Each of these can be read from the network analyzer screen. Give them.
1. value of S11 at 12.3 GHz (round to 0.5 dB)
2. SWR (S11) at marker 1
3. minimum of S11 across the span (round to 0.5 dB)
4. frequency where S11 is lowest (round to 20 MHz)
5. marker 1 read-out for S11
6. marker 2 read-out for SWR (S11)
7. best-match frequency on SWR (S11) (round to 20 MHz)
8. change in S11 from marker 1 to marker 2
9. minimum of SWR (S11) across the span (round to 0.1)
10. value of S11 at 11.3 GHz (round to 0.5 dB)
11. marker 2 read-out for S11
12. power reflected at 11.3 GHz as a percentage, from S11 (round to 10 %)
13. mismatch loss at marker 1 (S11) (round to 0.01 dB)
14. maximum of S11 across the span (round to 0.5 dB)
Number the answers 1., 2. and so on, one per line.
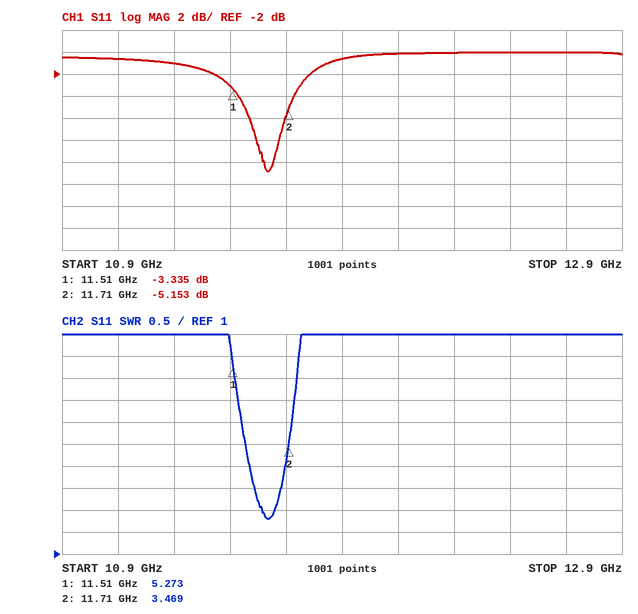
1. 0.0 dB
2. 5.273
3. -11.0 dB
4. 11.64 GHz
5. -3.335 dB
6. 3.469
7. 11.64 GHz
8. -1.818 dB
9. 1.8
10. -1.0 dB
11. -5.153 dB
12. 80 %
13. 2.71 dB
14. 0.0 dB
